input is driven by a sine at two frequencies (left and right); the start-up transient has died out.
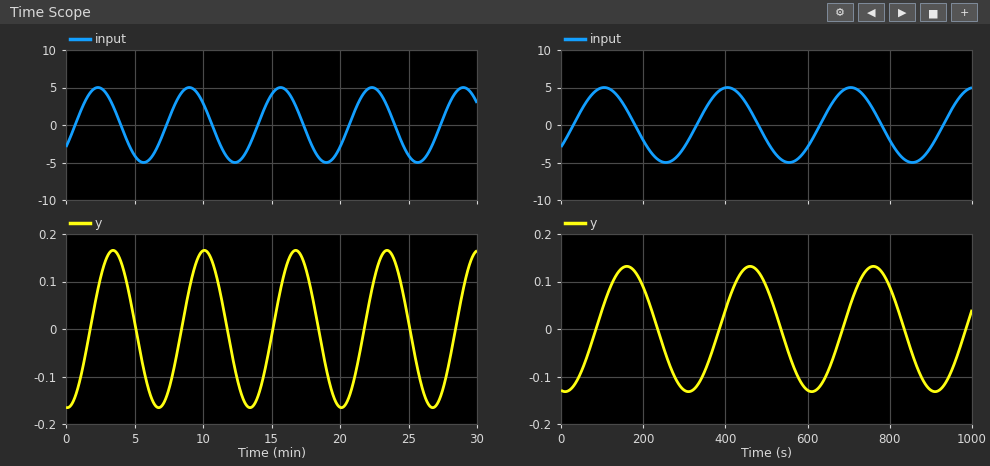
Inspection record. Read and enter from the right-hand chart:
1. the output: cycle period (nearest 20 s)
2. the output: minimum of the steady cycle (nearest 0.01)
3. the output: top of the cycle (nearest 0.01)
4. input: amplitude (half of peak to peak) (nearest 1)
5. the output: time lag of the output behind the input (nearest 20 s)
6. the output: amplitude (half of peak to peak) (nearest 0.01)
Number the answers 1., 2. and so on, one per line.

1. 300 s
2. -0.13
3. 0.13
4. 5
5. 60 s
6. 0.13
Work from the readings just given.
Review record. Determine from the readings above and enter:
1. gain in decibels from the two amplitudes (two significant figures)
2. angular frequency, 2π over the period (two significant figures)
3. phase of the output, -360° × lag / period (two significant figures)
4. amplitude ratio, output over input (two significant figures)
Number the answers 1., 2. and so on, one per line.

1. -32 dB
2. 0.021 rad/s
3. -72°
4. 0.026
